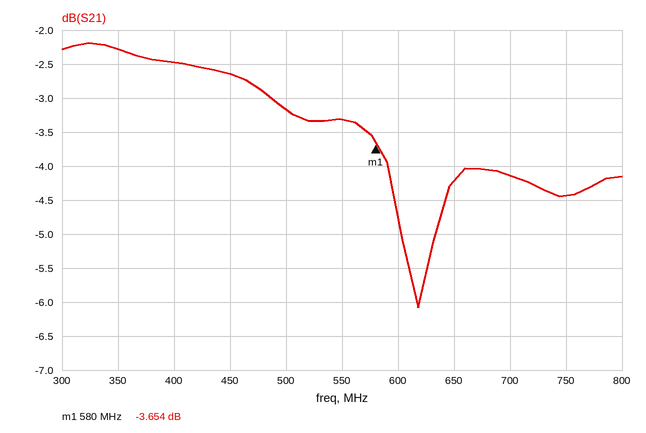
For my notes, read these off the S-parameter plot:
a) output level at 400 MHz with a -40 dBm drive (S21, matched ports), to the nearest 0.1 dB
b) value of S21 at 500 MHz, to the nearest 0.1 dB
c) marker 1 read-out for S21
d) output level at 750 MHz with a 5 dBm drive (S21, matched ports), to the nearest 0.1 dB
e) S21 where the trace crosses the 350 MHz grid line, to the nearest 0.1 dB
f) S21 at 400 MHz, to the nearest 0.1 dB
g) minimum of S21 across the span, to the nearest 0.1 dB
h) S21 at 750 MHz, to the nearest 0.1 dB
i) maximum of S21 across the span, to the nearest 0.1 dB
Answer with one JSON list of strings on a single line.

["-42.5 dBm", "-3.2 dB", "-3.654 dB", "0.6 dBm", "-2.3 dB", "-2.5 dB", "-6.1 dB", "-4.4 dB", "-2.2 dB"]
